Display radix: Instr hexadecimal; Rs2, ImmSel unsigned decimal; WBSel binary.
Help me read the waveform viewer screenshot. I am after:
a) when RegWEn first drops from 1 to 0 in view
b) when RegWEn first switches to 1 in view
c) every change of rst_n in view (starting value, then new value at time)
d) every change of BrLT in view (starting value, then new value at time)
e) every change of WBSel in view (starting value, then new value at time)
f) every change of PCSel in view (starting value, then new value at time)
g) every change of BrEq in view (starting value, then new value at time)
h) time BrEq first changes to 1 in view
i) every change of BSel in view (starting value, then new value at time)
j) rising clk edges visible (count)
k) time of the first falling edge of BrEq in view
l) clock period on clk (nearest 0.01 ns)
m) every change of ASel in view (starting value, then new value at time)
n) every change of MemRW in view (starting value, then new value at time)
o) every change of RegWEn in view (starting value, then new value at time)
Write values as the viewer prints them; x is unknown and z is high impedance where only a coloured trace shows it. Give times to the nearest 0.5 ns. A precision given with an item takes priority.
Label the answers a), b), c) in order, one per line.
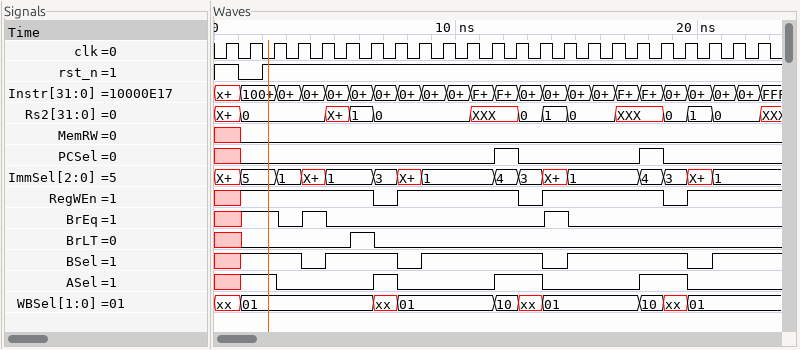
a) 6.5 ns
b) 1 ns
c) 1, 0 at 1 ns, 1 at 2 ns
d) x, 0 at 1 ns, 1 at 5.5 ns, 0 at 6.5 ns
e) xx, 01 at 1 ns, xx at 6.5 ns, 01 at 7.5 ns, 10 at 11.5 ns, xx at 12.5 ns, 01 at 13.5 ns, 10 at 17.5 ns, xx at 18.5 ns, 01 at 19.5 ns
f) x, 0 at 1 ns, 1 at 11.5 ns, 0 at 12.5 ns, 1 at 17.5 ns, 0 at 18.5 ns
g) x, 1 at 1 ns, 0 at 2.5 ns, 1 at 3.5 ns, 0 at 4.5 ns, 1 at 13.5 ns, 0 at 14.5 ns
h) 1 ns
i) x, 1 at 1 ns, 0 at 3.5 ns, 1 at 4.5 ns, 0 at 7.5 ns, 1 at 8.5 ns, 0 at 13.5 ns, 1 at 14.5 ns, 0 at 19.5 ns, 1 at 20.5 ns
j) 23
k) 2.5 ns
l) 1 ns
m) x, 1 at 1 ns, 0 at 2.5 ns, 1 at 6.5 ns, 0 at 7.5 ns, 1 at 11.5 ns, 0 at 13.5 ns, 1 at 17.5 ns, 0 at 19.5 ns
n) x, 0 at 1 ns
o) x, 1 at 1 ns, 0 at 6.5 ns, 1 at 7.5 ns, 0 at 12.5 ns, 1 at 13.5 ns, 0 at 18.5 ns, 1 at 19.5 ns
